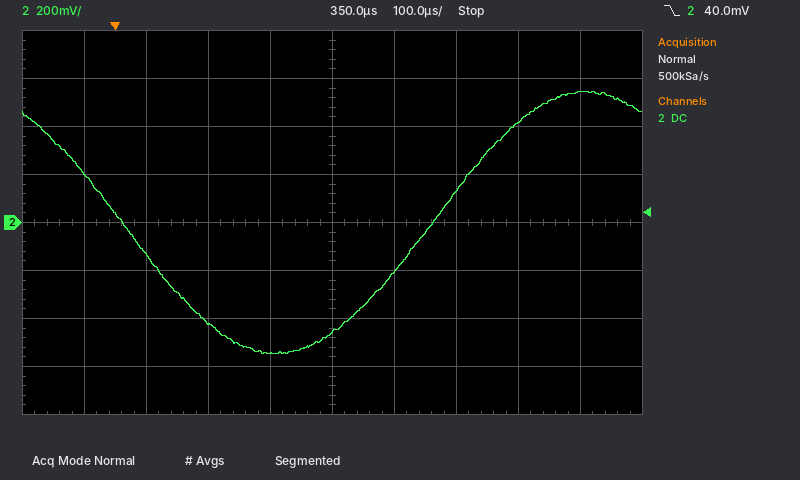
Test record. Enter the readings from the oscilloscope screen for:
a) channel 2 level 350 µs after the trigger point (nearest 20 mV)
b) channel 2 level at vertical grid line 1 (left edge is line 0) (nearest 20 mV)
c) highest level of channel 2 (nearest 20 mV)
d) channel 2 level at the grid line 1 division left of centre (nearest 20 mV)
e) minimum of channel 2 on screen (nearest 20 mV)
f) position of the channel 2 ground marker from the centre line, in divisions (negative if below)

-460 mV
200 mV
540 mV
-540 mV
-540 mV
0.0 div
